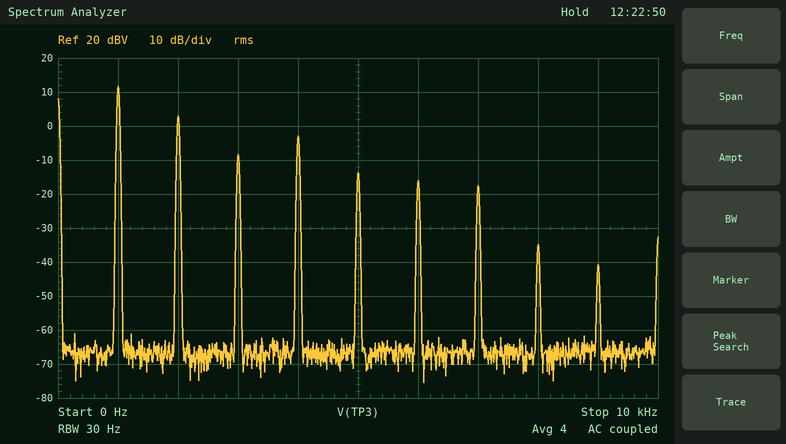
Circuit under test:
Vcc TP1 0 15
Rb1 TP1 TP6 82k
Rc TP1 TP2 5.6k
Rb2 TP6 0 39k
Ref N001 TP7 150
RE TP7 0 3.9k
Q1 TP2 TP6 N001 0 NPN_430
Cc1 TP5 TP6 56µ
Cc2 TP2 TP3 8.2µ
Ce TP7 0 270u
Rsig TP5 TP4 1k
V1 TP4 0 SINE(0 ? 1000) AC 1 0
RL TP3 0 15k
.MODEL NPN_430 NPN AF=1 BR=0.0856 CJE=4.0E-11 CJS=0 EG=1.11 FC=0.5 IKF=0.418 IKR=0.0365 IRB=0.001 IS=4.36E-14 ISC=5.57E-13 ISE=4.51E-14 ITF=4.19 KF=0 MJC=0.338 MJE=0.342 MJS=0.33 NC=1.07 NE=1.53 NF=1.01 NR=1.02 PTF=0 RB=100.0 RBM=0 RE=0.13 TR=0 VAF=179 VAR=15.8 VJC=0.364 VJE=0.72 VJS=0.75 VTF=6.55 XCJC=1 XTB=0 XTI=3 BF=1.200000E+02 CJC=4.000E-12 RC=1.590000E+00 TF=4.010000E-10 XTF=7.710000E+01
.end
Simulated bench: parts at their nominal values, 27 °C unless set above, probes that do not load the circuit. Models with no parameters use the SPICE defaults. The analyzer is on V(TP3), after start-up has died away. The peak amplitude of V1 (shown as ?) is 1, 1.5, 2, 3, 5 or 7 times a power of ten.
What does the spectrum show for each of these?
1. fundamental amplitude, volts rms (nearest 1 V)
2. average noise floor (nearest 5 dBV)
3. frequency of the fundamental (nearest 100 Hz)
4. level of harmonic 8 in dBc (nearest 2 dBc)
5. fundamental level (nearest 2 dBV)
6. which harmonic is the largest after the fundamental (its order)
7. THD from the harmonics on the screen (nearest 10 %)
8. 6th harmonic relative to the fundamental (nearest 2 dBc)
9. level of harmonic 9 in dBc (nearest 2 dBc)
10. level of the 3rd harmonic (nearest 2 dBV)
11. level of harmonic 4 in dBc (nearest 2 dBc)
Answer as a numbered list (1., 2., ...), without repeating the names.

1. 4 V
2. -65 dBV
3. 1.0 kHz
4. -46 dBc
5. 12 dBV
6. 2
7. 40 %
8. -28 dBc
9. -52 dBc
10. -8 dBV
11. -14 dBc
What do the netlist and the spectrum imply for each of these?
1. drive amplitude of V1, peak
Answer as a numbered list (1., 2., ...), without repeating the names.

1. 700 mV
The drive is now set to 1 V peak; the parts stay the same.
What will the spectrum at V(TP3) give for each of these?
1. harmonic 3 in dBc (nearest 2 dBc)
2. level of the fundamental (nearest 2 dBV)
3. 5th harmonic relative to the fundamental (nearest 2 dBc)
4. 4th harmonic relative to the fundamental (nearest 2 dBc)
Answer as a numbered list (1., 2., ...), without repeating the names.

1. -30 dBc
2. 12 dBV
3. -18 dBc
4. -14 dBc
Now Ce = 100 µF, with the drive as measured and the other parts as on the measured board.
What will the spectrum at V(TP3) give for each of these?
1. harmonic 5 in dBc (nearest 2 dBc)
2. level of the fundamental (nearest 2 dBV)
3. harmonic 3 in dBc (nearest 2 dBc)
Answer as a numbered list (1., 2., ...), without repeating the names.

1. -28 dBc
2. 12 dBV
3. -18 dBc
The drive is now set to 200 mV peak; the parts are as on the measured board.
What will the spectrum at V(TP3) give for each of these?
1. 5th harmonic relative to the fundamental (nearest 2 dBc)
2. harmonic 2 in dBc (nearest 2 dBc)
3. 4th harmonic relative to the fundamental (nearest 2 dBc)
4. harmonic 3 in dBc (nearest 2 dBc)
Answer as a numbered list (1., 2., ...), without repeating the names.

1. -58 dBc
2. -24 dBc
3. -46 dBc
4. -34 dBc
